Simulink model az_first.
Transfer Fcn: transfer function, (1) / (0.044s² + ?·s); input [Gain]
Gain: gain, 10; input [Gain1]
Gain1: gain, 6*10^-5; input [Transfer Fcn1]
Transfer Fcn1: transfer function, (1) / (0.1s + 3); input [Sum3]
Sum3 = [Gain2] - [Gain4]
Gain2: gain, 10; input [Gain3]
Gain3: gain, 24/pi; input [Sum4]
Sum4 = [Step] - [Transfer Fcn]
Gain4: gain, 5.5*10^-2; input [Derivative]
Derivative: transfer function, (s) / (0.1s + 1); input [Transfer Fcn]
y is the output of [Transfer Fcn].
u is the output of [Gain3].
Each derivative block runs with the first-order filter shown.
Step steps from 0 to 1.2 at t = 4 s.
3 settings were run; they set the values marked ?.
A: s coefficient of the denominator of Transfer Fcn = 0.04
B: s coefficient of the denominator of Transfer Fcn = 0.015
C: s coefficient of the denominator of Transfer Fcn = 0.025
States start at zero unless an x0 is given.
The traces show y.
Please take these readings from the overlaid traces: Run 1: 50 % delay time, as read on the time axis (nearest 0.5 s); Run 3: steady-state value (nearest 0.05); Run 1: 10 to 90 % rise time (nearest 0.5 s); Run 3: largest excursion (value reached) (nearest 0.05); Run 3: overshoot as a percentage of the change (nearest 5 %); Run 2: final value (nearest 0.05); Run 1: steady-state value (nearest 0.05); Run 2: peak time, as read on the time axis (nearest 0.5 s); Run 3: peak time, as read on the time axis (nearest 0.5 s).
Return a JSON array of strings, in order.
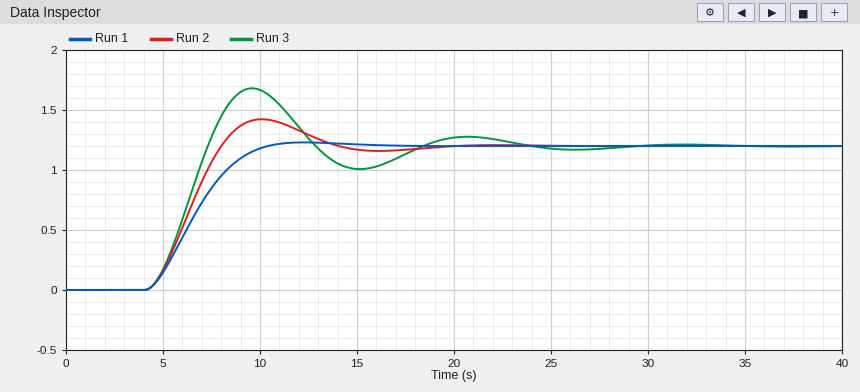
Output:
["6.5 s", "1.20", "4.0 s", "1.70", "40 %", "1.20", "1.20", "10.0 s", "9.5 s"]
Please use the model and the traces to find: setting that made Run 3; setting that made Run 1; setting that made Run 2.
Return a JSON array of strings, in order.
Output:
["B", "A", "C"]
